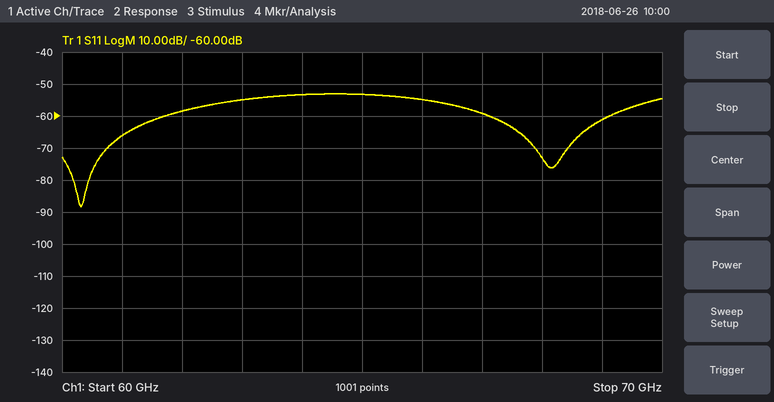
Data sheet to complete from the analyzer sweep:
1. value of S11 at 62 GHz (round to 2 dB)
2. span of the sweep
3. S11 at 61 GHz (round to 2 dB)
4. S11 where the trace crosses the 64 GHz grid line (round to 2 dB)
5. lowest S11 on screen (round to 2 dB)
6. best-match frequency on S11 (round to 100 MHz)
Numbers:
-58 dB
10 GHz
-66 dB
-54 dB
-88 dB
60.3 GHz
